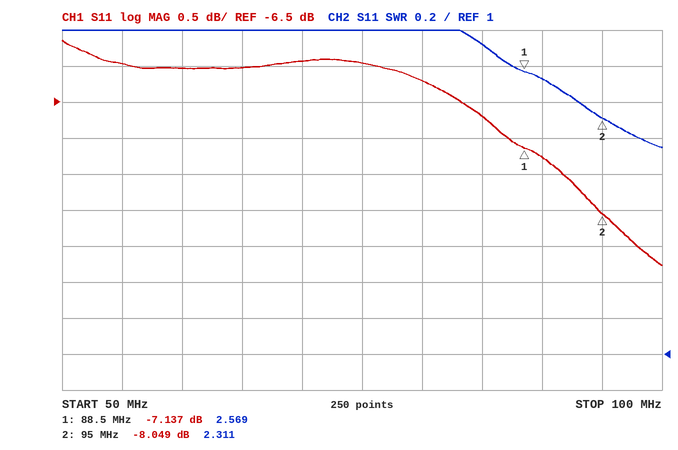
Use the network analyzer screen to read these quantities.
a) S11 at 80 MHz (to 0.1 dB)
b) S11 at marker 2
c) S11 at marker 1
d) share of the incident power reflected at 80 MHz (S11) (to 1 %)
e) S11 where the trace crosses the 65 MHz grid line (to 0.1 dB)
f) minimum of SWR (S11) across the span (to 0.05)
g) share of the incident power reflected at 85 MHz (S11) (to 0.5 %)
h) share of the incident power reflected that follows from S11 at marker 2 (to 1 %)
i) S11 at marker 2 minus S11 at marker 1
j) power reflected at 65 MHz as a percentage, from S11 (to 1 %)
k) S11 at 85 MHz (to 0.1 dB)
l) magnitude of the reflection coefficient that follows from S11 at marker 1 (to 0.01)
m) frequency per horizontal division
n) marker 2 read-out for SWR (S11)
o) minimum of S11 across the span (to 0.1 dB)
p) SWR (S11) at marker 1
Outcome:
-6.2 dB
-8.049 dB
-7.137 dB
24 %
-6.0 dB
2.15
21.5 %
16 %
-0.912 dB
25 %
-6.7 dB
0.44
5 MHz
2.311
-8.8 dB
2.569
